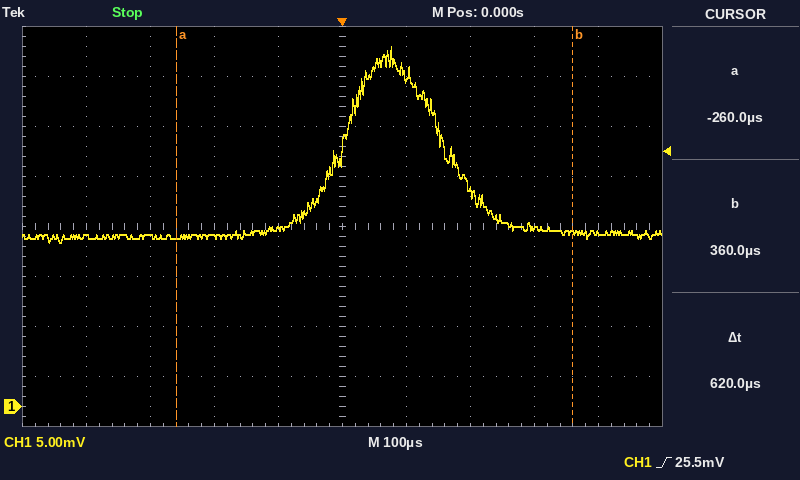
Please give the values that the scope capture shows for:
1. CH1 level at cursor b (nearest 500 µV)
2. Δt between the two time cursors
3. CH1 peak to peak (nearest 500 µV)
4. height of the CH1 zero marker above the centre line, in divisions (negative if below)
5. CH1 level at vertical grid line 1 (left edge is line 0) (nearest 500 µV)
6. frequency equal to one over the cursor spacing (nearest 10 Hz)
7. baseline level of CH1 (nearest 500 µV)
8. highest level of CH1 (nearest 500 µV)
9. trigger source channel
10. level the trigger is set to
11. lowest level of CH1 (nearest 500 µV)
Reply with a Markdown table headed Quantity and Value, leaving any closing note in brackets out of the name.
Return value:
| Quantity | Value |
|---|---|
| CH1 level at cursor b | 17.5 mV |
| Δt between the two time cursors | 620 µs |
| CH1 peak to peak | 19.5 mV |
| height of the CH1 zero marker above the centre line, in divisions | -3.6 div |
| CH1 level at vertical grid line 1 (left edge is line 0) | 17.0 mV |
| frequency equal to one over the cursor spacing | 1.61 kHz |
| baseline level of CH1 | 17.0 mV |
| highest level of CH1 | 36.0 mV |
| trigger source channel | CH1 |
| level the trigger is set to | 25.5 mV |
| lowest level of CH1 | 16.5 mV |
